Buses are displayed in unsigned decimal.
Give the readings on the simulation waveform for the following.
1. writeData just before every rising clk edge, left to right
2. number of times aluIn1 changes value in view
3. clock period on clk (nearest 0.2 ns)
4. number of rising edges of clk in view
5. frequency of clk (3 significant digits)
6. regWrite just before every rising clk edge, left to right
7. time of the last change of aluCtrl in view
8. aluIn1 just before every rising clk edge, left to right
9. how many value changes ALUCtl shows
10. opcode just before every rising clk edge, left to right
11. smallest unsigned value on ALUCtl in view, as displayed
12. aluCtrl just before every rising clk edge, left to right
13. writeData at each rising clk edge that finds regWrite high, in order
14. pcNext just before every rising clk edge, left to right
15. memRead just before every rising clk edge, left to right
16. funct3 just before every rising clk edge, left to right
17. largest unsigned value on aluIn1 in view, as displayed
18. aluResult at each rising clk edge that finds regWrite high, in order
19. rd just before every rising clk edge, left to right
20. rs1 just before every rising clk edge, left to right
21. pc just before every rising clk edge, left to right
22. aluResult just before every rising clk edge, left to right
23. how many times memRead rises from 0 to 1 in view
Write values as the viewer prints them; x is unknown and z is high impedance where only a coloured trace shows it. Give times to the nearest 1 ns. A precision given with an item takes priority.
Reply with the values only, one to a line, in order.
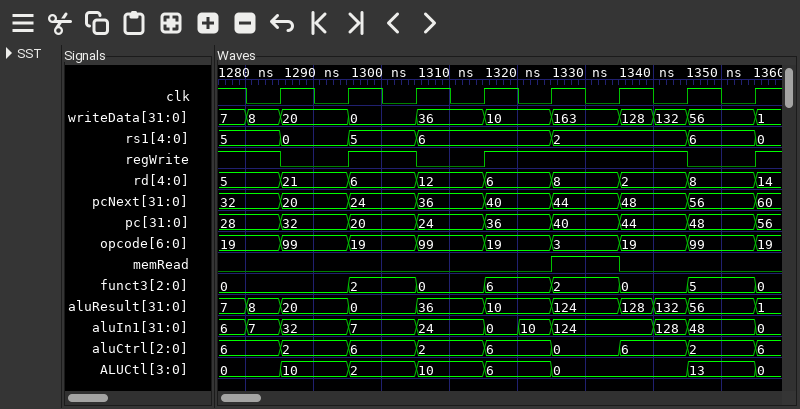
8, 20, 0, 36, 10, 163, 132, 56
10
10 ns
8
100 MHz
1 0 1 0 1 1 1 0
1355 ns
7, 32, 7, 24, 10, 124, 128, 48
7
19, 99, 19, 99, 19, 3, 19, 99
0
6, 2, 6, 2, 6, 0, 6, 2
8, 0, 10, 163, 132
32, 20, 24, 36, 40, 44, 48, 56
0 0 0 0 0 1 0 0
0, 0, 2, 0, 6, 2, 0, 5
128
8, 0, 10, 124, 132
5, 21, 6, 12, 6, 8, 2, 8
5, 0, 5, 6, 6, 2, 2, 6
28, 32, 20, 24, 36, 40, 44, 48
8, 20, 0, 36, 10, 124, 132, 56
1
